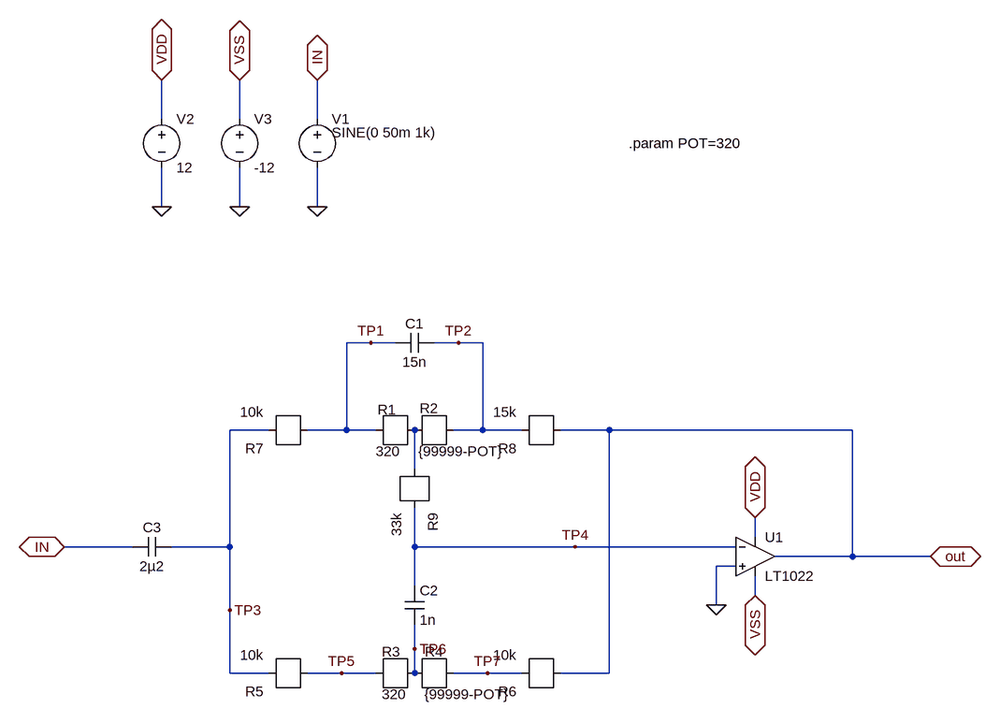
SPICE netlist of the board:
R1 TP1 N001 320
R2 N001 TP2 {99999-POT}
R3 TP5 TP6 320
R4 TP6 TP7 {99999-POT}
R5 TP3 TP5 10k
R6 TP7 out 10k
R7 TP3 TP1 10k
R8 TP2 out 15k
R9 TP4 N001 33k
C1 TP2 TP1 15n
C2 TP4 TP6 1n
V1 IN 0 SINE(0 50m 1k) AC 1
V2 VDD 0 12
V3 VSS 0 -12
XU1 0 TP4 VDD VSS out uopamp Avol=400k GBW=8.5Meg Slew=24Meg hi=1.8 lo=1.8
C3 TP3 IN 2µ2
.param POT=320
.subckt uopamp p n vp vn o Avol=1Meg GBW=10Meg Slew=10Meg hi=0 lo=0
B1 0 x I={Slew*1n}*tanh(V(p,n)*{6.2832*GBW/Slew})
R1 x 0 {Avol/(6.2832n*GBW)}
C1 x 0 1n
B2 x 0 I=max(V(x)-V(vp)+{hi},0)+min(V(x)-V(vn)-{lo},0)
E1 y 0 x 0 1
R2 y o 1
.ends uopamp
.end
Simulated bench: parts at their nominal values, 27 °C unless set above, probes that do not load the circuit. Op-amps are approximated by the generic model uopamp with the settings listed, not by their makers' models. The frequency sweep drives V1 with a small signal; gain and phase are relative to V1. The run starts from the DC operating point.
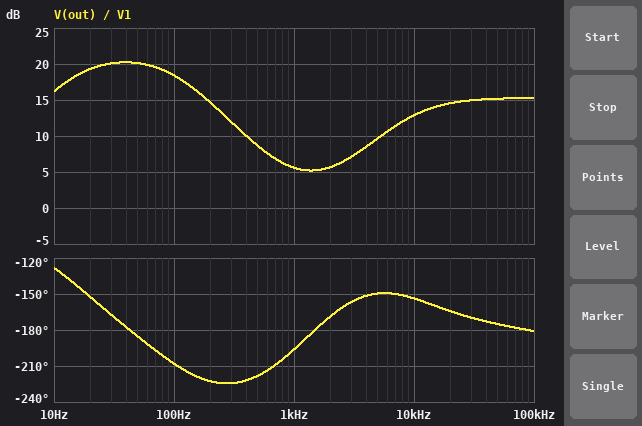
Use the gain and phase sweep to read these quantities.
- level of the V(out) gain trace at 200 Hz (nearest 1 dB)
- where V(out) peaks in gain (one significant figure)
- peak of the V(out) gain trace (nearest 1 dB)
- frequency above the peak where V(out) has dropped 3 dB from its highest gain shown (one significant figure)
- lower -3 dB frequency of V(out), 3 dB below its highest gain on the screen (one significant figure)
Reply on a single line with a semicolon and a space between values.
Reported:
15 dB; 40 Hz; 20 dB; 100 Hz; 10 Hz
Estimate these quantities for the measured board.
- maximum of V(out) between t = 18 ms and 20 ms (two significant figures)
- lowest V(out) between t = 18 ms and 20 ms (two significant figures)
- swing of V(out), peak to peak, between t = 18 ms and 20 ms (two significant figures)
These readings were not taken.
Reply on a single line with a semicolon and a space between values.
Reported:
97 mV; -94 mV; 190 mV
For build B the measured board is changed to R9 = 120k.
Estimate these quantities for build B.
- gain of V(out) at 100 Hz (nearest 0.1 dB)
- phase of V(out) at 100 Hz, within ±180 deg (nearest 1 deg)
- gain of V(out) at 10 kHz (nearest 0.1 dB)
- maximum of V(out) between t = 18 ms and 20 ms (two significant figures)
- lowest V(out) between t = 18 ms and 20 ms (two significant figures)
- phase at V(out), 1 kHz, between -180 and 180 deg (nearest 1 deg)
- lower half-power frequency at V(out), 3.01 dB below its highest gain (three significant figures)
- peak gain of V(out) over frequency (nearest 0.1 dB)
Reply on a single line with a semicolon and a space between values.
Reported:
18.2 dB; 153 deg; 17.5 dB; 120 mV; -120 mV; -171 deg; 11.9 Hz; 20.2 dB
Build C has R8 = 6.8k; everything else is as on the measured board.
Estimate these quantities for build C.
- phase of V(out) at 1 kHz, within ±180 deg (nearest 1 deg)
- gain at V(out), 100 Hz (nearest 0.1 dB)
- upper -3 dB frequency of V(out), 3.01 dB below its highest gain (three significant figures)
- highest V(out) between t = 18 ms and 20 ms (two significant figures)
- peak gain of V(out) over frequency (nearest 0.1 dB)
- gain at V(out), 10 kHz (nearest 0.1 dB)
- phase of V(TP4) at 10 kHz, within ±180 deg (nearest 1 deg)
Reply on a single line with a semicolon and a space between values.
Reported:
147 deg; 17.7 dB; 127 Hz; 63 mV; 19.6 dB; 9.3 dB; 123 deg
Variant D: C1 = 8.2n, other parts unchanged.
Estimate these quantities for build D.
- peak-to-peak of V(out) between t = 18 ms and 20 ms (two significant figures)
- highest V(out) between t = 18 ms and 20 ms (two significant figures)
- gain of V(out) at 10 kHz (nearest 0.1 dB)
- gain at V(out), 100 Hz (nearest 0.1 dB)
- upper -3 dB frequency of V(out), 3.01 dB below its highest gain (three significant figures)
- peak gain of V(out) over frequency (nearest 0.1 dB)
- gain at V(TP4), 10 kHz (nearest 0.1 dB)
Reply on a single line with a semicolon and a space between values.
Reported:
250 mV; 130 mV; 12.8 dB; 20.0 dB; 216 Hz; 20.5 dB; -45.8 dB
